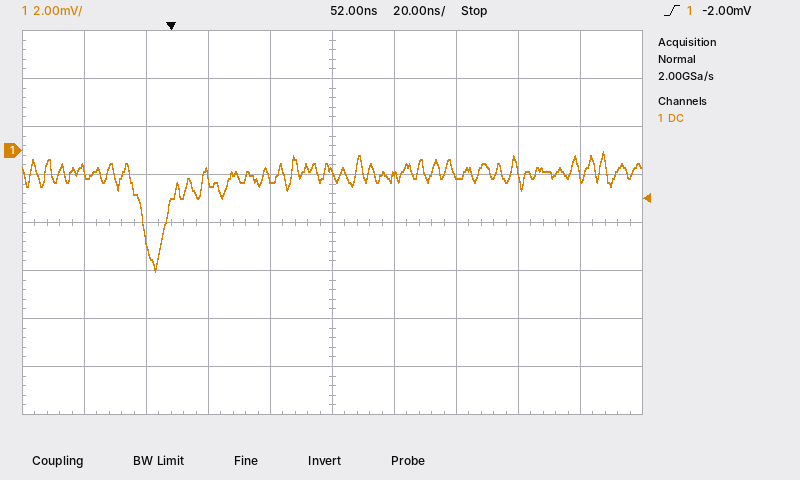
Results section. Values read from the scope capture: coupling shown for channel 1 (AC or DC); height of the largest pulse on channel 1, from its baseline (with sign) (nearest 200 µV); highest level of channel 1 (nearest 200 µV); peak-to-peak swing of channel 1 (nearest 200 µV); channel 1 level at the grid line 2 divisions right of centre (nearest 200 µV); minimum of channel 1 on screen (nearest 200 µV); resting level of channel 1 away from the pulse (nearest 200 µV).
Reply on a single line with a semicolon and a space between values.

DC; -4.0 mV; 0.0 mV; 5.0 mV; -1.0 mV; -5.0 mV; -1.0 mV
